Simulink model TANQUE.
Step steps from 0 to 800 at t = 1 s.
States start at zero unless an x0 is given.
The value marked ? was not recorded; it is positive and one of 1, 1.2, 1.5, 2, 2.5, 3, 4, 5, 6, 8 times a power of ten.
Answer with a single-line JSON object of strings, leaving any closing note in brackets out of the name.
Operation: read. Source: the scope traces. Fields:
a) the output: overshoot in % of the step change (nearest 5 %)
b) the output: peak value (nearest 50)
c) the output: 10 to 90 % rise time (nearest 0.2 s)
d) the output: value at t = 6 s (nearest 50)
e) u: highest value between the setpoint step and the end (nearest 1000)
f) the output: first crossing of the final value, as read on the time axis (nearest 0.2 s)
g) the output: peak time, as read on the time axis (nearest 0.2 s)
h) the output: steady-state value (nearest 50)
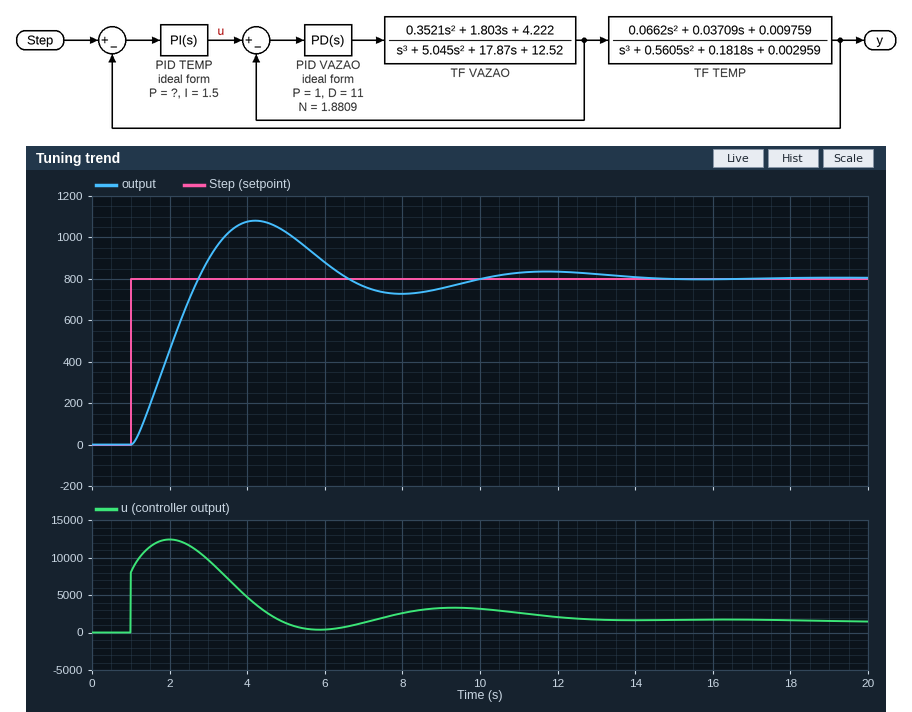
{"the output: overshoot in % of the step change": "35 %", "the output: peak value": "1100", "the output: 10 to 90 % rise time": "1.2 s", "the output: value at t = 6 s": "900", "u: highest value between the setpoint step and the end": "12000", "the output: first crossing of the final value, as read on the time axis": "2.8 s", "the output: peak time, as read on the time axis": "4.2 s", "the output: steady-state value": "800"}
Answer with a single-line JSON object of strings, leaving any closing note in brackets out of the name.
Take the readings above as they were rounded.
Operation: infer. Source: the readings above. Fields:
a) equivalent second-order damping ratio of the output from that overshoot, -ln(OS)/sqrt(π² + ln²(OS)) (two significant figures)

{"equivalent second-order damping ratio of the output from that overshoot, -ln(OS)/sqrt(π² + ln²(OS))": "0.32"}
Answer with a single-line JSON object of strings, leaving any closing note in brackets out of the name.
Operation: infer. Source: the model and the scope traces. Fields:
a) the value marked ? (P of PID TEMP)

{"the value marked ?": "10"}
